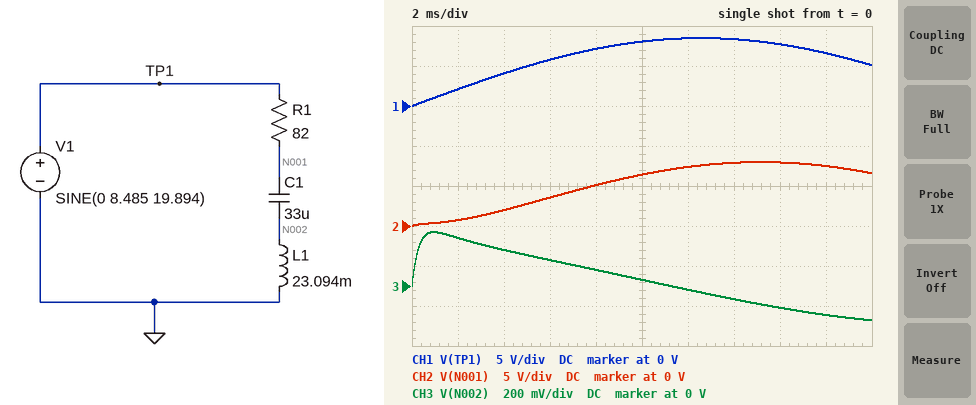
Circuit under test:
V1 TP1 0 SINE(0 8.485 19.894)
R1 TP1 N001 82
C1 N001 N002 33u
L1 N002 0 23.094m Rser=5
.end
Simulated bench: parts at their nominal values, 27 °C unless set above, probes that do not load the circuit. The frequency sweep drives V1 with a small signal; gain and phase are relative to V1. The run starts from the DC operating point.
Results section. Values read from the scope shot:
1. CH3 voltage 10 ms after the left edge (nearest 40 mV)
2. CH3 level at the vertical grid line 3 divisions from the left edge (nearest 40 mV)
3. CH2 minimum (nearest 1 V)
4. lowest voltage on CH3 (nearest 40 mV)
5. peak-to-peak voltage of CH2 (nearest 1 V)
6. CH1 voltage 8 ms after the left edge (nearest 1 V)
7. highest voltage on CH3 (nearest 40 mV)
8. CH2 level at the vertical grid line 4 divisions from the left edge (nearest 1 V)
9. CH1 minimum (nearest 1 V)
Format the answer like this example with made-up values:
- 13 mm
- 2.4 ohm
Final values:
- 40 mV
- 120 mV
- 0 V
- -160 mV
- 8 V
- 7 V
- 280 mV
- 5 V
- 0 V
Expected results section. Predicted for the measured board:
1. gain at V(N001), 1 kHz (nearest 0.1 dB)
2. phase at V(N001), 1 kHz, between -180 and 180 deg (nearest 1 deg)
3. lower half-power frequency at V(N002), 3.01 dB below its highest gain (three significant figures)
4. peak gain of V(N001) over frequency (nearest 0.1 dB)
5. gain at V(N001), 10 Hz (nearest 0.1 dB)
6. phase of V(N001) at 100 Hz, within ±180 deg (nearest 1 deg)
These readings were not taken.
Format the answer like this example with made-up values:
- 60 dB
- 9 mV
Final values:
- -1.4 dB
- 30 deg
- 543 Hz
- 0 dB
- -0.1 dB
- -60 deg
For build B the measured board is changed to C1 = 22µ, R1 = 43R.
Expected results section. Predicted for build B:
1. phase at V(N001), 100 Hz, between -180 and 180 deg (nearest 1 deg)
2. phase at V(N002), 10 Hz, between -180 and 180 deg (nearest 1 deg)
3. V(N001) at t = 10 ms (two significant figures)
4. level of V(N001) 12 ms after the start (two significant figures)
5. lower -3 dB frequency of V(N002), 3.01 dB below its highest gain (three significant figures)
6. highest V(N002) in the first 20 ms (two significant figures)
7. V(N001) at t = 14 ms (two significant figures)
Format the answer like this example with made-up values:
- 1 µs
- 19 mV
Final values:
- -35 deg
- 102 deg
- 7.6 V
- 8.3 V
- 232 Hz
- 380 mV
- 8.4 V
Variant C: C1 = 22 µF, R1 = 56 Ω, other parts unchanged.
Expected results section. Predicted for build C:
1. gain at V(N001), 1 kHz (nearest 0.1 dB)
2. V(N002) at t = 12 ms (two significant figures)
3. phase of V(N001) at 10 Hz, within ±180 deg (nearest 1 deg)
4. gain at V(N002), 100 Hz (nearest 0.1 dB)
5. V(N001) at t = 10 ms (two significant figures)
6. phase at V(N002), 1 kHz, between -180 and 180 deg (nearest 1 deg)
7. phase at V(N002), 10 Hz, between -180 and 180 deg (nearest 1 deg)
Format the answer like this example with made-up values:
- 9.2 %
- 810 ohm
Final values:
- -0.8 dB
- -38 mV
- -4 deg
- -14.8 dB
- 7.4 V
- 22 deg
- 101 deg
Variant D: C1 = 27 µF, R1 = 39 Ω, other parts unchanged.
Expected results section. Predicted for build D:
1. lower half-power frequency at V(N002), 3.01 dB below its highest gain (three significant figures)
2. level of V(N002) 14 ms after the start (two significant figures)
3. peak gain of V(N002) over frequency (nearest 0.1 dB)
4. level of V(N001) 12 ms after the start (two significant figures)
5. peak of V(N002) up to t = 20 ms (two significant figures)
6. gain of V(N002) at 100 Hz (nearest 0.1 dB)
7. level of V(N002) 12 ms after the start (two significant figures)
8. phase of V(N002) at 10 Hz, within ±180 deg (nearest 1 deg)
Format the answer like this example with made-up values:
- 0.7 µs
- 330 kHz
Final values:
- 212 Hz
- -87 mV
- 0 dB
- 8.2 V
- 420 mV
- -12.2 dB
- -49 mV
- 102 deg
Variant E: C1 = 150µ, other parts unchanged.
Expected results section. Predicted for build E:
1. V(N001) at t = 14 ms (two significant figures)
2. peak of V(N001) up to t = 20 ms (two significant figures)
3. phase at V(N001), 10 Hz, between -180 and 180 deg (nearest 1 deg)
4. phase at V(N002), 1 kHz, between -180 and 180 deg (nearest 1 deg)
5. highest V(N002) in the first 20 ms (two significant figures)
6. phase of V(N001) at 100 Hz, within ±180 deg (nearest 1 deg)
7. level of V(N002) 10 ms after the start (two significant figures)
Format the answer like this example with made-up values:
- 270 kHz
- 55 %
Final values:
- 4.3 V
- 5.1 V
- -37 deg
- 29 deg
- 390 mV
- 35 deg
- 300 mV
